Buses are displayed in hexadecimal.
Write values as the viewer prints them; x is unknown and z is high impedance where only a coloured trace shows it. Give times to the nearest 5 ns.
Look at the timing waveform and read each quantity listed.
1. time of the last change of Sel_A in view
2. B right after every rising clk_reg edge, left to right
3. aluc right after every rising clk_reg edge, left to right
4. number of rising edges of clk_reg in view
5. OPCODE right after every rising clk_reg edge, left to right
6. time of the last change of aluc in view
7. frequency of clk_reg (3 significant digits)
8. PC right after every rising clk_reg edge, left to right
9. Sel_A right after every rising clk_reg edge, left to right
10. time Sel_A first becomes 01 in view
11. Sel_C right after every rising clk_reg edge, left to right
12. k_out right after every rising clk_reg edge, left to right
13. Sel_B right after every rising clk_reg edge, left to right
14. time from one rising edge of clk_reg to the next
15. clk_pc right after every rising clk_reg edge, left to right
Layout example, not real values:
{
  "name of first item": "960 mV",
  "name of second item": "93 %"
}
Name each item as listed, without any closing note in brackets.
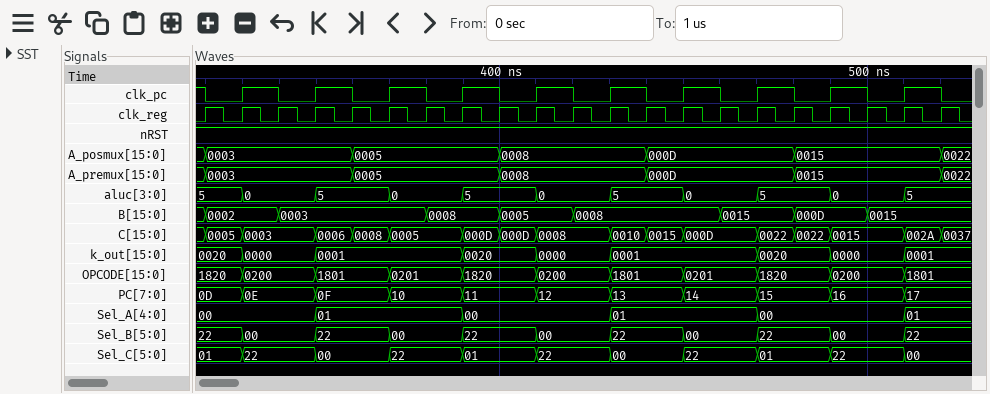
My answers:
{
  "time of the last change of Sel_A in view": "510 ns",
  "B right after every rising clk_reg edge, left to right": "0002, 0002, 0003, 0003, 0003, 0003, 0008, 0008, 0005, 0005, 0008, 0008, 0008, 0008, 0015, 0015, 000D, 000D, 0015, 0015, 0015",
  "aluc right after every rising clk_reg edge, left to right": "5, 0, 0, 5, 5, 0, 0, 5, 5, 0, 0, 5, 5, 0, 0, 5, 5, 0, 0, 5, 5",
  "number of rising edges of clk_reg in view": "21",
  "OPCODE right after every rising clk_reg edge, left to right": "1820, 0200, 0200, 1801, 1801, 0201, 0201, 1820, 1820, 0200, 0200, 1801, 1801, 0201, 0201, 1820, 1820, 0200, 0200, 1801, 1801",
  "time of the last change of aluc in view": "510 ns",
  "frequency of clk_reg": "100 MHz",
  "PC right after every rising clk_reg edge, left to right": "0D, 0E, 0E, 0F, 0F, 10, 10, 11, 11, 12, 12, 13, 13, 14, 14, 15, 15, 16, 16, 17, 17",
  "Sel_A right after every rising clk_reg edge, left to right": "00, 00, 00, 01, 01, 01, 01, 00, 00, 00, 00, 01, 01, 01, 01, 00, 00, 00, 00, 01, 01",
  "time Sel_A first becomes 01 in view": "350 ns",
  "Sel_C right after every rising clk_reg edge, left to right": "01, 22, 22, 00, 00, 22, 22, 01, 01, 22, 22, 00, 00, 22, 22, 01, 01, 22, 22, 00, 00",
  "k_out right after every rising clk_reg edge, left to right": "0020, 0000, 0000, 0001, 0001, 0001, 0001, 0020, 0020, 0000, 0000, 0001, 0001, 0001, 0001, 0020, 0020, 0000, 0000, 0001, 0001",
  "Sel_B right after every rising clk_reg edge, left to right": "22, 00, 00, 22, 22, 00, 00, 22, 22, 00, 00, 22, 22, 00, 00, 22, 22, 00, 00, 22, 22",
  "time from one rising edge of clk_reg to the next": "10 ns",
  "clk_pc right after every rising clk_reg edge, left to right": "0 1 0 1 0 1 0 1 0 1 0 1 0 1 0 1 0 1 0 1 0"
}
